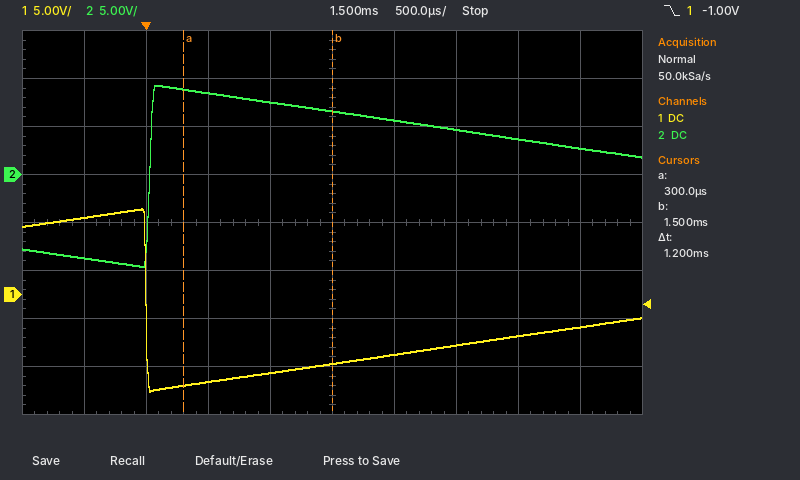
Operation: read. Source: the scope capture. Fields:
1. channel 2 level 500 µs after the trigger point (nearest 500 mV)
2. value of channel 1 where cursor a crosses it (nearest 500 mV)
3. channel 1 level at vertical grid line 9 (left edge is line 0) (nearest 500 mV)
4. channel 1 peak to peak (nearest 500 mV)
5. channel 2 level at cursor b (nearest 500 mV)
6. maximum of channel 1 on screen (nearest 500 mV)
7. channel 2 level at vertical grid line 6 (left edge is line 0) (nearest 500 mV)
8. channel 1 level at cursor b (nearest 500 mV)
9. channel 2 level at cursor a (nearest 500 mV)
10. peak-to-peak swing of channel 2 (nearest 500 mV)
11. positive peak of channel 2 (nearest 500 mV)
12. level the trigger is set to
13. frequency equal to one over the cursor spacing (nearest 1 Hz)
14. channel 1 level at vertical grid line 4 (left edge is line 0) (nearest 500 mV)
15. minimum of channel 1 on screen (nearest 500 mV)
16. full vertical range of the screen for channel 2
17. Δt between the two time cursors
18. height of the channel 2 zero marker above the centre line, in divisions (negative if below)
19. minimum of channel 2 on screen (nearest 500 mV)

8.5 V
-9.5 V
-3.5 V
19.0 V
6.5 V
9.0 V
5.5 V
-7.0 V
9.0 V
19.0 V
9.5 V
-1.00 V
833 Hz
-8.0 V
-10.0 V
40 V
1.2 ms
+1.0 div
-9.5 V
